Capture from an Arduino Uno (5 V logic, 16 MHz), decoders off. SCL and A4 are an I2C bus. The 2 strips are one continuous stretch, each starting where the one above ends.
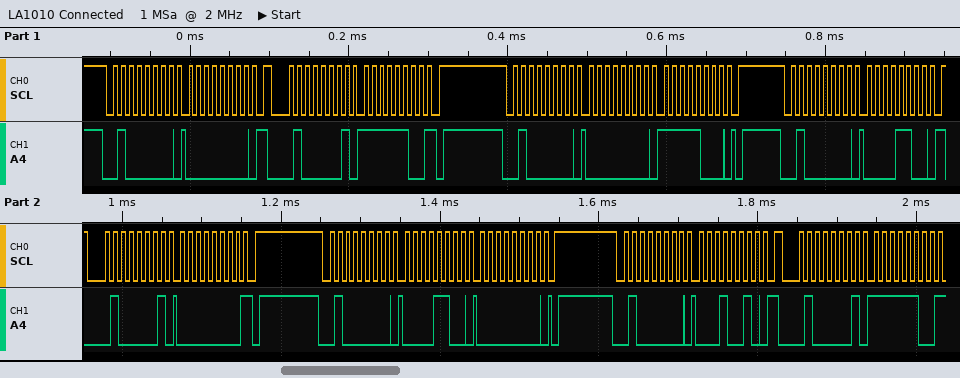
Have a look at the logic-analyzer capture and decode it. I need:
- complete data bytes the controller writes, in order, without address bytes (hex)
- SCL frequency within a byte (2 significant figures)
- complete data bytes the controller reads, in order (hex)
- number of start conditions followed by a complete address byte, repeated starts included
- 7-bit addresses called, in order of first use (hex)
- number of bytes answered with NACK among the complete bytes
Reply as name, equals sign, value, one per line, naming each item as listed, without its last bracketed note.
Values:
complete data bytes the controller writes, in order, without address bytes = 00 00 F8 0C 0C 00 12
SCL frequency within a byte = 100 kHz
complete data bytes the controller reads, in order = FC 00 FC
number of start conditions followed by a complete address byte, repeated starts included = 8
7-bit addresses called, in order of first use = 0x20
number of bytes answered with NACK among the complete bytes = 3
